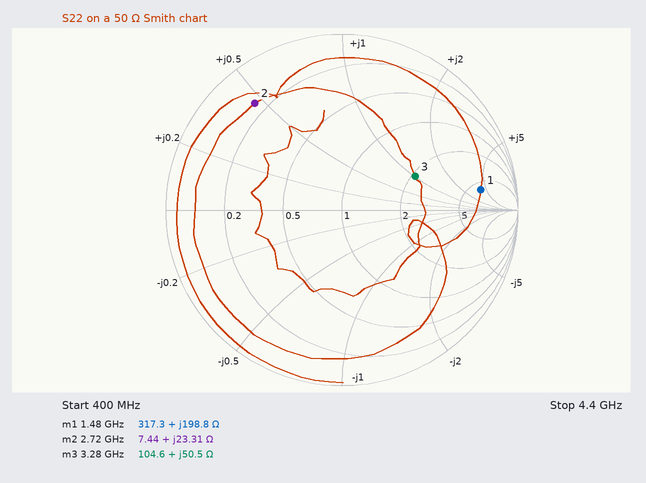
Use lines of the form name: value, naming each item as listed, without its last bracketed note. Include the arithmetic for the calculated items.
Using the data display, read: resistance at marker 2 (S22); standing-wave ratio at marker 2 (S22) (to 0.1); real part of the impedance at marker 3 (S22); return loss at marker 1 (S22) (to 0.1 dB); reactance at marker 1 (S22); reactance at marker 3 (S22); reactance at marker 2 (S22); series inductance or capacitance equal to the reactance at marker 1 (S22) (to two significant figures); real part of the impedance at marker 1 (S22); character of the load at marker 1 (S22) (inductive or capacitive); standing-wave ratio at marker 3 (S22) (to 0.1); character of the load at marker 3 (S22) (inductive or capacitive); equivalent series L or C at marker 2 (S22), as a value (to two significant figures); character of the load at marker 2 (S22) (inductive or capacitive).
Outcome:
resistance at marker 2: 7.44 Ω
standing-wave ratio at marker 2 (S22): 8.2
real part of the impedance at marker 3: 104.6 Ω
return loss at marker 1 (S22): 2.0 dB
reactance at marker 1: +198.8 Ω
reactance at marker 3: +50.5 Ω
reactance at marker 2: +23.31 Ω
series inductance or capacitance equal to the reactance at marker 1 (S22): L = 198.8 Ω/(2π × 1.48 GHz) ≈ 21 nH
real part of the impedance at marker 1: 317.3 Ω
character of the load at marker 1 (S22): inductive
standing-wave ratio at marker 3 (S22): 2.7
character of the load at marker 3 (S22): inductive
equivalent series L or C at marker 2 (S22), as a value: L = 23.31 Ω/(2π × 2.72 GHz) ≈ 1.4 nH
character of the load at marker 2 (S22): inductive
